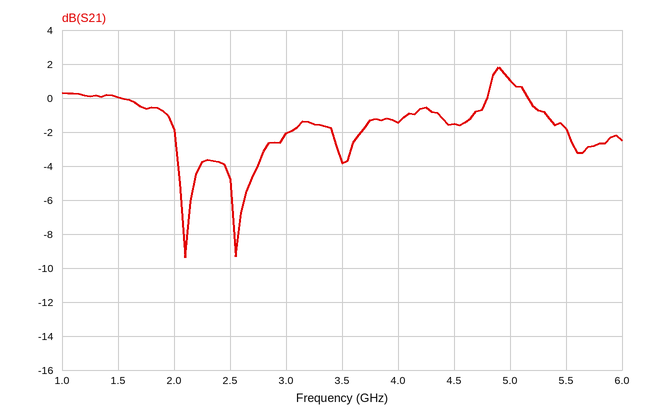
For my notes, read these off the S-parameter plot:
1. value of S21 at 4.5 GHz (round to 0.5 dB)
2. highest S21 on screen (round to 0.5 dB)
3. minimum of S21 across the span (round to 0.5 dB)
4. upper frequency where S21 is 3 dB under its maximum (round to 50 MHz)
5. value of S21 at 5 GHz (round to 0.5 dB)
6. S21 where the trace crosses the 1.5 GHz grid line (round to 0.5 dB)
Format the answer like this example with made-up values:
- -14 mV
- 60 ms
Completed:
- -1.5 dB
- 2.0 dB
- -9.5 dB
- 5.35 GHz
- 1.0 dB
- 0.0 dB
